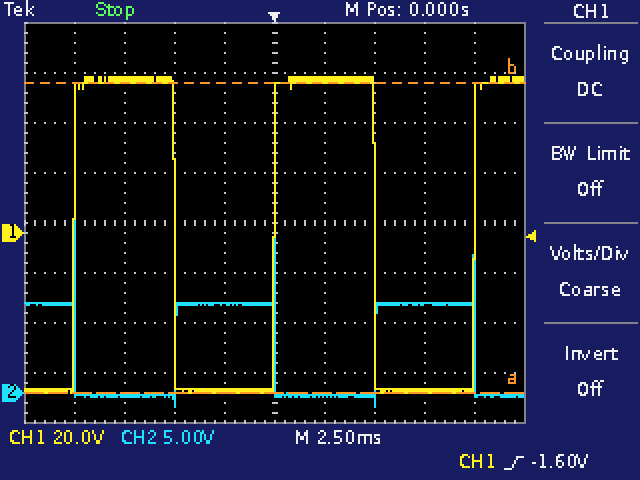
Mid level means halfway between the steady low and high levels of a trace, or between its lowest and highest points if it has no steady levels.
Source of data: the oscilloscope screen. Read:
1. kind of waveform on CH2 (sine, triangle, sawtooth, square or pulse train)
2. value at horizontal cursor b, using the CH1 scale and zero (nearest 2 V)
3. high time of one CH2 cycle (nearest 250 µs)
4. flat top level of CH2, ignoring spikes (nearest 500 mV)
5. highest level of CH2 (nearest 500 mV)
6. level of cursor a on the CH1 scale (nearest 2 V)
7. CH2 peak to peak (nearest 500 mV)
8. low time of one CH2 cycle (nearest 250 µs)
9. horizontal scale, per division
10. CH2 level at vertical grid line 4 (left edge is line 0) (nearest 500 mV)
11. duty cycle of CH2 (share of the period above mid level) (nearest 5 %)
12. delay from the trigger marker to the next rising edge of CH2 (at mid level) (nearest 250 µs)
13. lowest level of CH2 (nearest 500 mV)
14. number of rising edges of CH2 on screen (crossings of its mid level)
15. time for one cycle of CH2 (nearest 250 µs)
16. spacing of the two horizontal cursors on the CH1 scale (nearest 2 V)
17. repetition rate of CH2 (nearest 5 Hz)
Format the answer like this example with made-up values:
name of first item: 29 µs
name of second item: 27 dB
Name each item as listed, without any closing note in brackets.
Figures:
kind of waveform on CH2: square
value at horizontal cursor b, using the CH1 scale and zero: 60 V
high time of one CH2 cycle: 5.00 ms
flat top level of CH2, ignoring spikes: 9.0 V
highest level of CH2: 17.0 V
level of cursor a on the CH1 scale: -64 V
CH2 peak to peak: 18.5 V
low time of one CH2 cycle: 5.00 ms
horizontal scale, per division: 2.5 ms
CH2 level at vertical grid line 4 (left edge is line 0): 9.0 V
duty cycle of CH2 (share of the period above mid level): 50 %
delay from the trigger marker to the next rising edge of CH2 (at mid level): 5.00 ms
lowest level of CH2: -1.5 V
number of rising edges of CH2 on screen: 2
time for one cycle of CH2: 10.00 ms
spacing of the two horizontal cursors on the CH1 scale: 124 V
repetition rate of CH2: 100 Hz
